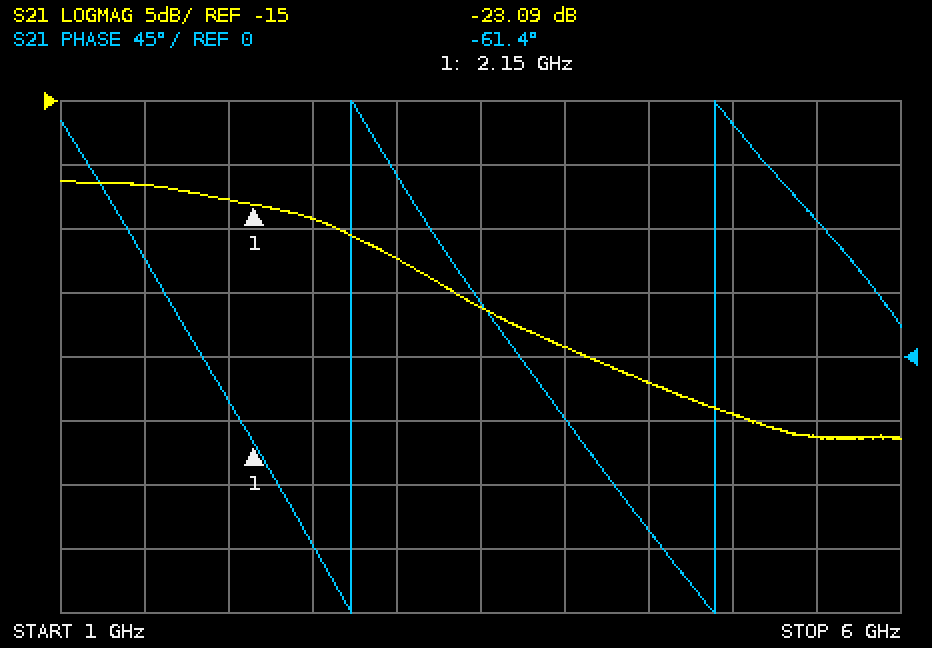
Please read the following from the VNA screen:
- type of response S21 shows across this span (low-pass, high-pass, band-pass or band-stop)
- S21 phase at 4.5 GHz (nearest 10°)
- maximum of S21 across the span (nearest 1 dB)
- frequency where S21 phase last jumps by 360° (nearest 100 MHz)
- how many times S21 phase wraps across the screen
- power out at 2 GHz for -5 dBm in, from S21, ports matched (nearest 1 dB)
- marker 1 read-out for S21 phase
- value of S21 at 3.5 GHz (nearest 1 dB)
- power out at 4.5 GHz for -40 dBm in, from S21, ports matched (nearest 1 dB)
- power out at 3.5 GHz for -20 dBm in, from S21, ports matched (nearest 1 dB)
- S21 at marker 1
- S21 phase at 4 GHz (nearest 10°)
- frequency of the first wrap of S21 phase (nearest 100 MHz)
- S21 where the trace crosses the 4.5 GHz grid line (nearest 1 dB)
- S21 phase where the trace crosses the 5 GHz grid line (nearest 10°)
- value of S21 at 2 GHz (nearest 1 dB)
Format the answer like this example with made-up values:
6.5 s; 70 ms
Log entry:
low-pass; -120°; -21 dB; 4.9 GHz; 2; -28 dBm; -61.4°; -31 dB; -77 dBm; -51 dBm; -23.09 dB; -40°; 2.7 GHz; -37 dB; 160°; -23 dB
